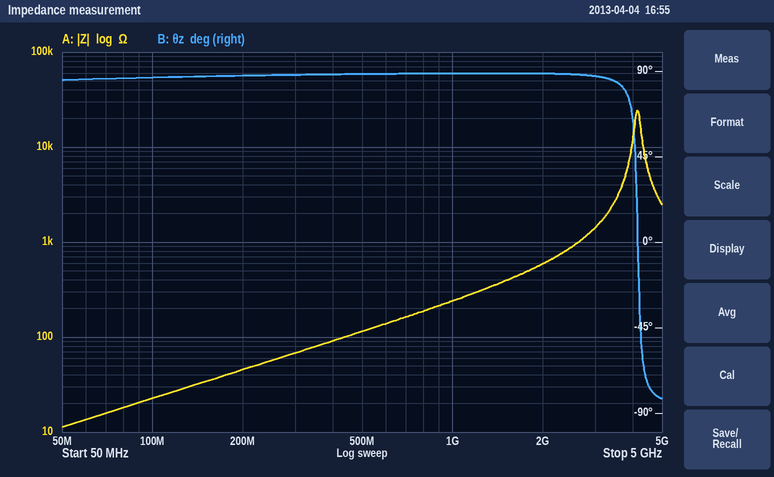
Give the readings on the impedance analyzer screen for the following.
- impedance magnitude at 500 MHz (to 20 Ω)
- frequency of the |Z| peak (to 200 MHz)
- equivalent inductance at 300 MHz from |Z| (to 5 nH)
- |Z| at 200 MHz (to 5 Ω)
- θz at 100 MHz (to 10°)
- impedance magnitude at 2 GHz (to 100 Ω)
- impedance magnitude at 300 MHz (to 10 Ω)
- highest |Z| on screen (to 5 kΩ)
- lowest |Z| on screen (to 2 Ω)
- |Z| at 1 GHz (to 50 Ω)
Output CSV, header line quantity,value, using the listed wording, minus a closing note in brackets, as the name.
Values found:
quantity,value
impedance magnitude at 500 MHz,120 Ω
frequency of the |Z| peak,4.2 GHz
equivalent inductance at 300 MHz from |Z|,35 nH
|Z| at 200 MHz,45 Ω
θz at 100 MHz,90°
impedance magnitude at 2 GHz,600 Ω
impedance magnitude at 300 MHz,70 Ω
highest |Z| on screen,25 kΩ
lowest |Z| on screen,12 Ω
|Z| at 1 GHz,250 Ω
